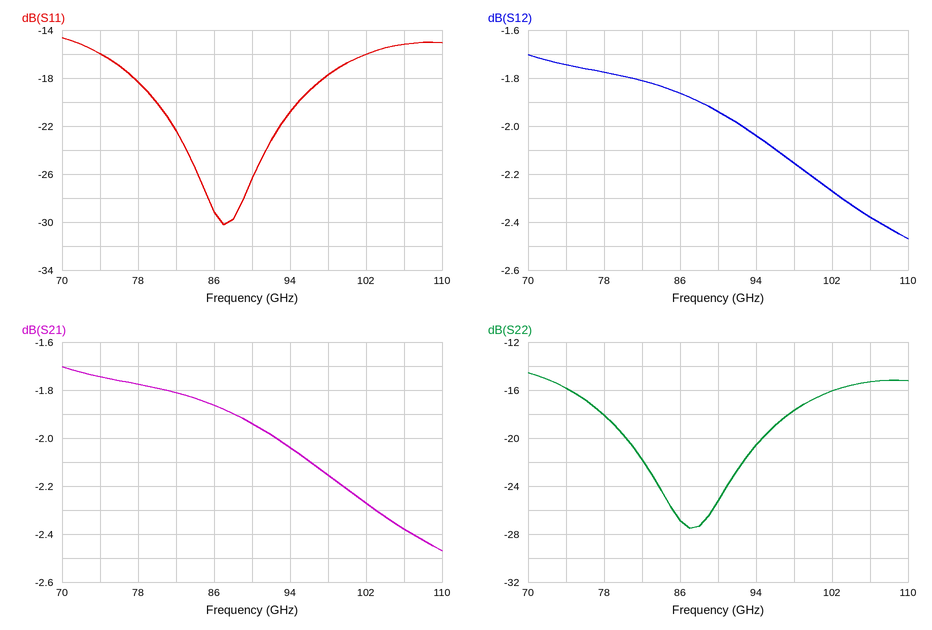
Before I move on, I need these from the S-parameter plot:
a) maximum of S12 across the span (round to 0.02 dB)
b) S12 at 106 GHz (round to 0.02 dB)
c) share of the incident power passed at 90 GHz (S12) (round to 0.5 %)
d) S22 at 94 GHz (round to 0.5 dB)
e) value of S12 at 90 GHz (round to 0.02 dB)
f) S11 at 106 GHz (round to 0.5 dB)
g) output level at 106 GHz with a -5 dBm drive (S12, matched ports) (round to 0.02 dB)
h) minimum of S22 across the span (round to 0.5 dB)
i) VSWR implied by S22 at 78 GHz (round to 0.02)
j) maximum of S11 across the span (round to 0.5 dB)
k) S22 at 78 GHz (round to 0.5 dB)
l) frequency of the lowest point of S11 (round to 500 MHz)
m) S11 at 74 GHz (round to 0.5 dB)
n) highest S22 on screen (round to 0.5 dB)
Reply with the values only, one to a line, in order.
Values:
-1.70 dB
-2.38 dB
64.0 %
-20.5 dB
-1.94 dB
-15.0 dB
-7.38 dBm
-27.5 dB
1.28
-14.5 dB
-18.0 dB
87.0 GHz
-16.0 dB
-14.5 dB
